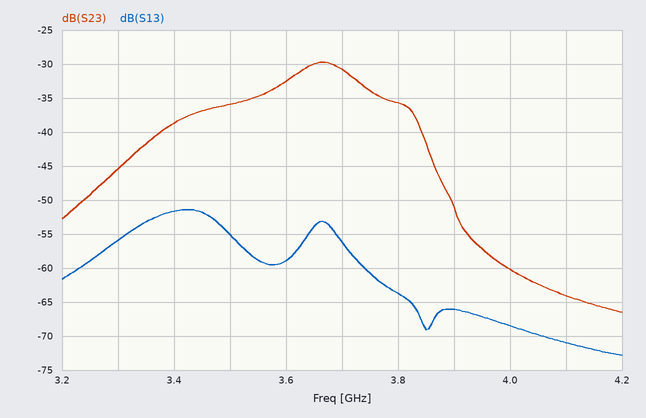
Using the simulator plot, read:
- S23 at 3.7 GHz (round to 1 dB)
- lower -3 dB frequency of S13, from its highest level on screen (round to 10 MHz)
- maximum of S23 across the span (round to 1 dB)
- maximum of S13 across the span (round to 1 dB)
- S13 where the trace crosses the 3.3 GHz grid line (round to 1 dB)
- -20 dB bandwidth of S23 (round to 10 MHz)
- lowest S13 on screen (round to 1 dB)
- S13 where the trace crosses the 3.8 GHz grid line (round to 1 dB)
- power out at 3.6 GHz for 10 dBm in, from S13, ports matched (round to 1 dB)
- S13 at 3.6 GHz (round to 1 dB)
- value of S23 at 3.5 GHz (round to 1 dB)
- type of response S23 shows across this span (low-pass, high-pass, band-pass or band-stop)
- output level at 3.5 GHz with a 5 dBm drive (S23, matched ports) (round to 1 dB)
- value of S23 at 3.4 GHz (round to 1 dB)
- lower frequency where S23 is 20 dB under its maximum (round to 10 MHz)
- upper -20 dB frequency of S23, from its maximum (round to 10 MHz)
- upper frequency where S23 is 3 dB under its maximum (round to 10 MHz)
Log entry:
-31 dB
3.33 GHz
-30 dB
-51 dB
-56 dB
650 MHz
-73 dB
-64 dB
-49 dBm
-59 dB
-36 dB
band-pass
-31 dBm
-39 dB
3.24 GHz
3.89 GHz
3.73 GHz
